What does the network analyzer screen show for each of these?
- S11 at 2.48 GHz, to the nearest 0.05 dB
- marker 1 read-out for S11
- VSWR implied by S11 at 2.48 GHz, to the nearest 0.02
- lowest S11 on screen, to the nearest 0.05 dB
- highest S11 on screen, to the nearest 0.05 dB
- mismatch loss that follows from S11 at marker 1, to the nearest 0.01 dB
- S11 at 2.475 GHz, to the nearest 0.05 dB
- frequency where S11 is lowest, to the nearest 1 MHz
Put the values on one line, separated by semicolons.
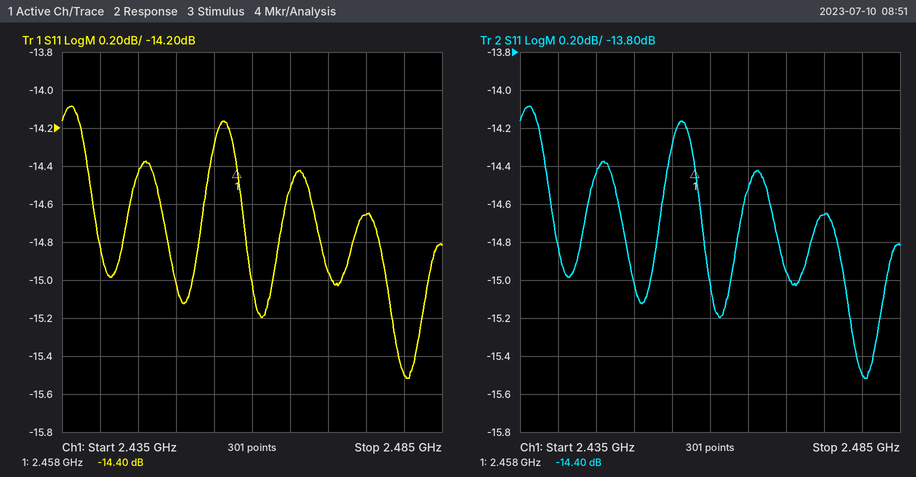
-15.50 dB; -14.40 dB; 1.40; -15.50 dB; -14.10 dB; 0.16 dB; -14.65 dB; 2.480 GHz
